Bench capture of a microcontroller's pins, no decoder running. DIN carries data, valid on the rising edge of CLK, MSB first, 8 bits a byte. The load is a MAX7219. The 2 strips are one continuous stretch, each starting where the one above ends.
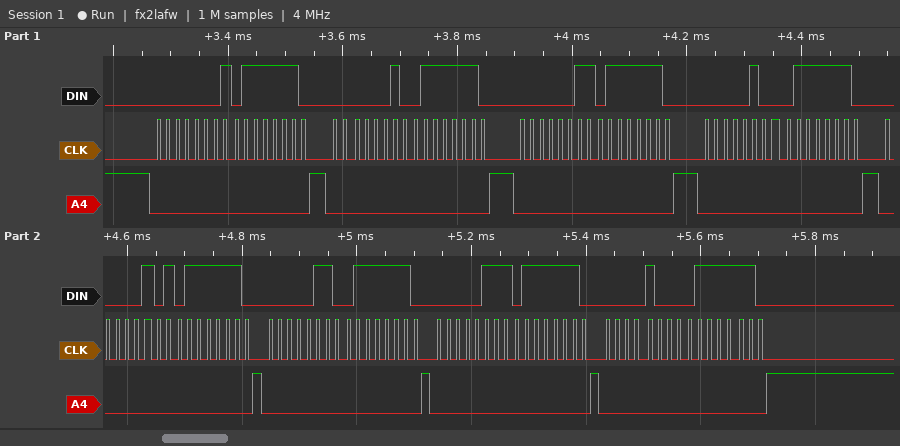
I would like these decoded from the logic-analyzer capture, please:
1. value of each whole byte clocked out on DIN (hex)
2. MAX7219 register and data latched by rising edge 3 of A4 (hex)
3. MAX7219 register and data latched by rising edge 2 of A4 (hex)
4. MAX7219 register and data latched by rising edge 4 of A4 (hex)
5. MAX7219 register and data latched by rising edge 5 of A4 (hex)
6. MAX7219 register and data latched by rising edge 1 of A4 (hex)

01 7E 02 7E 03 7E 04 7E 05 7E 06 7E 07 7E 08 7E
register 0x3, data 0x7E
register 0x2, data 0x7E
register 0x4, data 0x7E
register 0x5, data 0x7E
register 0x1, data 0x7E
